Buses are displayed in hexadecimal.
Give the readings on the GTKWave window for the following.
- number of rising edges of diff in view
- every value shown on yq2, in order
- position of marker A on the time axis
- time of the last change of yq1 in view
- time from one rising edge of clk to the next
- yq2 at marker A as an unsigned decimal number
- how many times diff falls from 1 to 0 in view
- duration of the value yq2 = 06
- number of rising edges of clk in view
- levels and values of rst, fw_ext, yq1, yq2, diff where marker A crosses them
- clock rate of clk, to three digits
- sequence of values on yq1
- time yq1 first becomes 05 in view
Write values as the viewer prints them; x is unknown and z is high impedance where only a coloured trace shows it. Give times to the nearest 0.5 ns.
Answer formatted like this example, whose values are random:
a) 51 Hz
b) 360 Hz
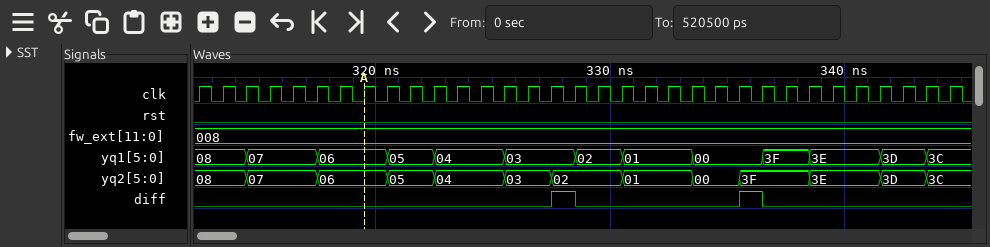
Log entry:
a) 2
b) 08, 07, 06, 05, 04, 03, 02, 01, 00, 3F, 3E, 3D, 3C
c) 319.5 ns
d) 343.5 ns
e) 1 ns
f) 6
g) 2
h) 3 ns
i) 33
j) rst=0, fw_ext=008, yq1=06, yq2=06, diff=0
k) 1.00 GHz
l) 08, 07, 06, 05, 04, 03, 02, 01, 00, 3F, 3E, 3D, 3C
m) 320.5 ns
